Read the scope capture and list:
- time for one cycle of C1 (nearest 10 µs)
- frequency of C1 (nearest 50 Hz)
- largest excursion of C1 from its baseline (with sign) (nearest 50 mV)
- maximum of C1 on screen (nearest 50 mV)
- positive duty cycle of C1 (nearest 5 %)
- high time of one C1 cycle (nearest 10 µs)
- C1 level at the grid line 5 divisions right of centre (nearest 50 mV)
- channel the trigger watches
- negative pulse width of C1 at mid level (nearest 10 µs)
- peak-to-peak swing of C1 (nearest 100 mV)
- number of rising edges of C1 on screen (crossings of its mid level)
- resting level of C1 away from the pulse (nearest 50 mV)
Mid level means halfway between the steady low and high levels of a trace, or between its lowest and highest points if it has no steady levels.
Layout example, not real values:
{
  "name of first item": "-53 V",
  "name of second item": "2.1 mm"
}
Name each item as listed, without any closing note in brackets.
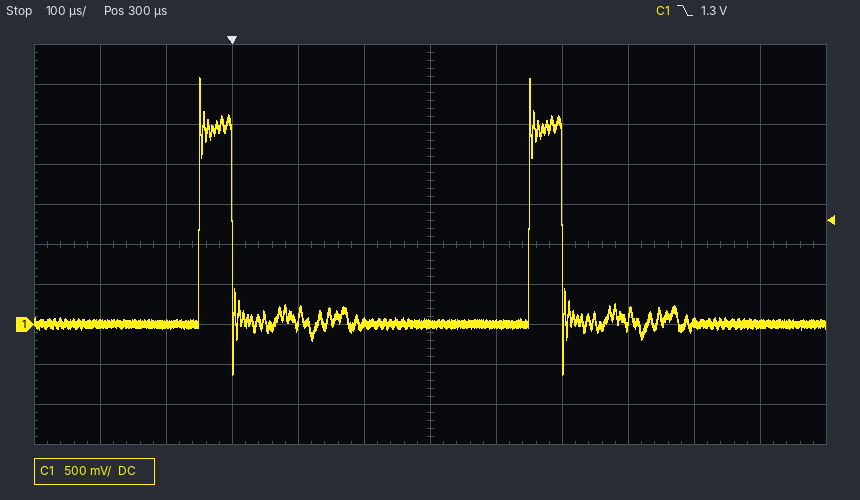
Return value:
{
  "time for one cycle of C1": "500 µs",
  "frequency of C1": "2.00 kHz",
  "largest excursion of C1 from its baseline (with sign)": "+3.10 V",
  "maximum of C1 on screen": "3.10 V",
  "positive duty cycle of C1": "10 %",
  "high time of one C1 cycle": "50 µs",
  "C1 level at the grid line 5 divisions right of centre": "0 mV",
  "channel the trigger watches": "C1",
  "negative pulse width of C1 at mid level": "450 µs",
  "peak-to-peak swing of C1": "3.70 V",
  "number of rising edges of C1 on screen": "2",
  "resting level of C1 away from the pulse": "0 mV"
}
